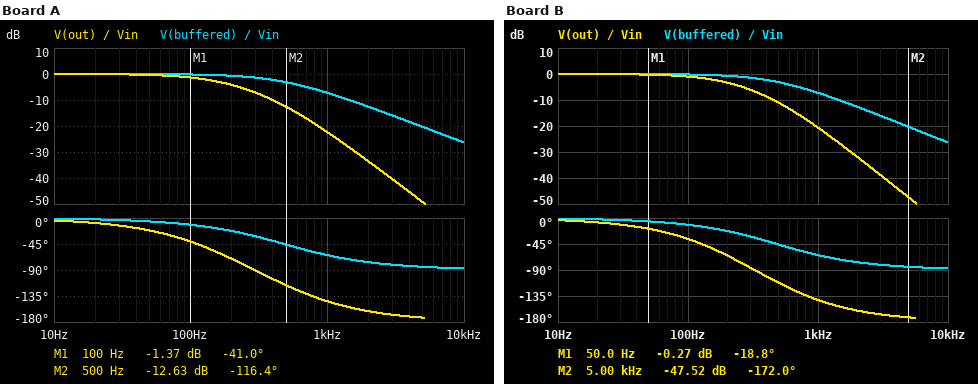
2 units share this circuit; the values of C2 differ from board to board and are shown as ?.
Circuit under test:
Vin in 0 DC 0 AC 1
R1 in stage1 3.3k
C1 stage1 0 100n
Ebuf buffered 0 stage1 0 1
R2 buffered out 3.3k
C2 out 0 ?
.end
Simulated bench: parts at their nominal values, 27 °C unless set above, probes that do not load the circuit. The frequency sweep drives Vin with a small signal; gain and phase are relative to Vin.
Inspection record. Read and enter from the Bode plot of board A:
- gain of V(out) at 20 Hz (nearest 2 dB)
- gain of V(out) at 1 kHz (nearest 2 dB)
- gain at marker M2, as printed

0 dB
-22 dB
-12.63 dB
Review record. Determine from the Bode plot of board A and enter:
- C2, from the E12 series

270 nF
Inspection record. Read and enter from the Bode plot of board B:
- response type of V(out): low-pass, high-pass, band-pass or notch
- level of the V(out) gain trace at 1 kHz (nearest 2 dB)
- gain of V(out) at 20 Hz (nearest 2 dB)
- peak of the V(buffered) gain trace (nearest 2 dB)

low-pass
-20 dB
0 dB
0 dB
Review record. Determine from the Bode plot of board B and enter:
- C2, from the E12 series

220 nF
